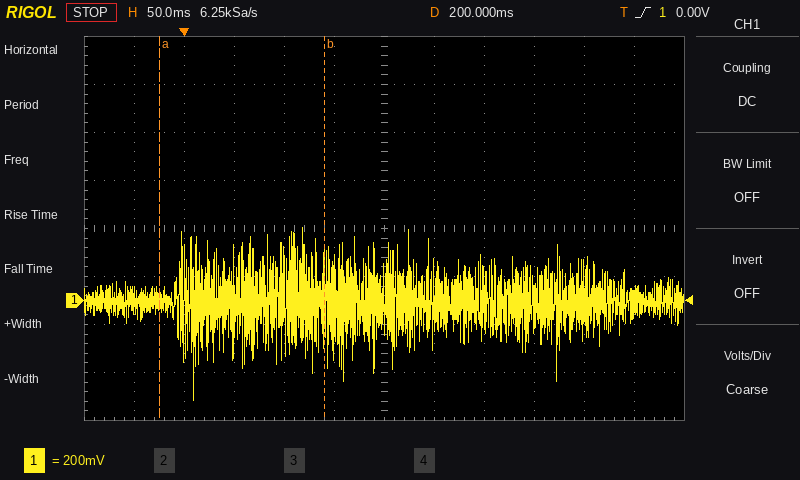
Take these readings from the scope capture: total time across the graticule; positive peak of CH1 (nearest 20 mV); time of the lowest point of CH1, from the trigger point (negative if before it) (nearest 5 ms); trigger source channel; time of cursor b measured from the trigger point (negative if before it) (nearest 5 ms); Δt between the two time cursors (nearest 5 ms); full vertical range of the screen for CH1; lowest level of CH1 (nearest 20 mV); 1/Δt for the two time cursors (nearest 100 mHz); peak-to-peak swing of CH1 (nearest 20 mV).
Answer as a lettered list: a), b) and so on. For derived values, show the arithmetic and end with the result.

a) 600 ms
b) 300 mV
c) +10 ms
d) CH1
e) +140 ms
f) 165 ms
g) 1.6 V
h) -420 mV
i) 1 / 165 ms ≈ 6.1 Hz
j) 300 mV − (-420 mV) = 720 mV
